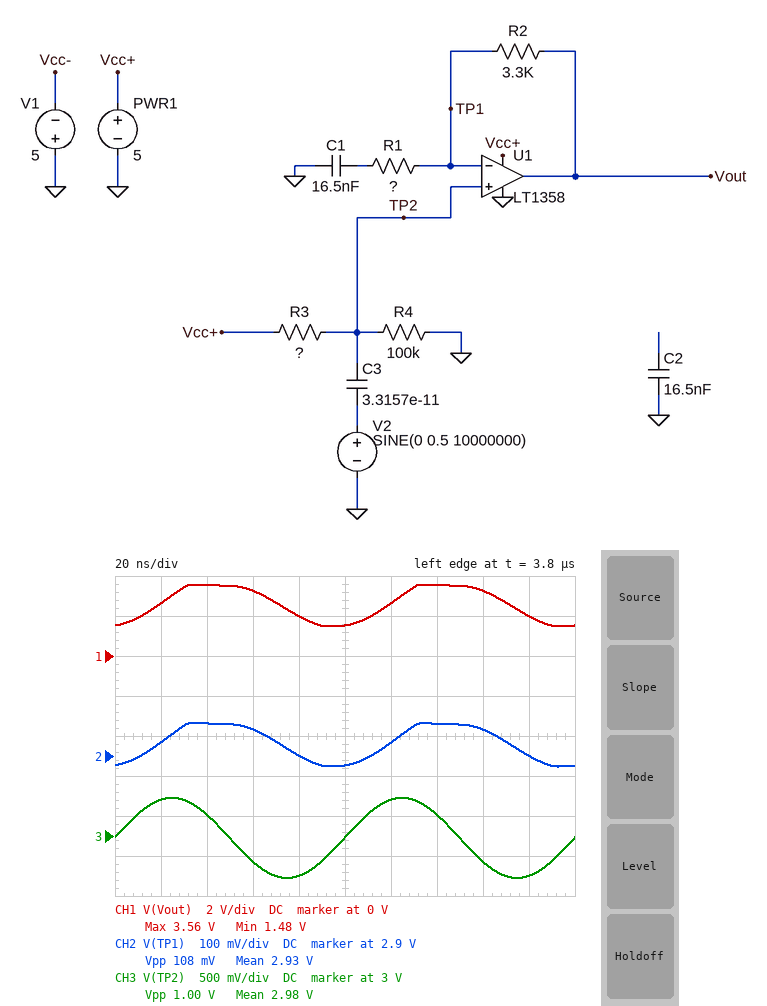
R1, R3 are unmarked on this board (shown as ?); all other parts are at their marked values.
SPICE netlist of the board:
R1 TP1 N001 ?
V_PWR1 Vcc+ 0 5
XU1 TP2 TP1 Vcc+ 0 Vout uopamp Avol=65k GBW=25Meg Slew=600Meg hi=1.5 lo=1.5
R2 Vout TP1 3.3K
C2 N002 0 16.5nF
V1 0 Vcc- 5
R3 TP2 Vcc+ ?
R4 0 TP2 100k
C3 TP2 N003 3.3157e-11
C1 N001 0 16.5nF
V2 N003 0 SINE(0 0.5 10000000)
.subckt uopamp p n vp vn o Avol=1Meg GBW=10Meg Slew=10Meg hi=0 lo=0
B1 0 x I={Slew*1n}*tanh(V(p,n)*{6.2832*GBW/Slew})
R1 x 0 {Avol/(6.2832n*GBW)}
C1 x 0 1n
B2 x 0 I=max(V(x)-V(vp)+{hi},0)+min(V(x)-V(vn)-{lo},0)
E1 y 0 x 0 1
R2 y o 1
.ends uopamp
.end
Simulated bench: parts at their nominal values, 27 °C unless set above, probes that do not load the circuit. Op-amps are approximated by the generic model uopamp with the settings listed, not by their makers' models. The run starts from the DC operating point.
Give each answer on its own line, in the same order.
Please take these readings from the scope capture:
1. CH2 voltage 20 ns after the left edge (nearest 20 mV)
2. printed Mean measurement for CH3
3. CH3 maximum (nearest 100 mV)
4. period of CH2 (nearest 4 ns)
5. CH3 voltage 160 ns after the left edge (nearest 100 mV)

2.94 V
2.98 V
3.5 V
100 ns
2.7 V
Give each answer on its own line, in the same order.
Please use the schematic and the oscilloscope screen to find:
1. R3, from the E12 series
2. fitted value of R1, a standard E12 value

68 kΩ
180 Ω
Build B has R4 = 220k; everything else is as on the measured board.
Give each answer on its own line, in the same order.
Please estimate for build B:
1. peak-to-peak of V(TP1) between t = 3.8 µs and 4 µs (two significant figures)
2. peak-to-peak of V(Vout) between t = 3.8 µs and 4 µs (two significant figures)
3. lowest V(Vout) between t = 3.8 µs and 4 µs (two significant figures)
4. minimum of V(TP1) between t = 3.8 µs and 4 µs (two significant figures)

37 mV
710 mV
2.9 V
3.5 V
